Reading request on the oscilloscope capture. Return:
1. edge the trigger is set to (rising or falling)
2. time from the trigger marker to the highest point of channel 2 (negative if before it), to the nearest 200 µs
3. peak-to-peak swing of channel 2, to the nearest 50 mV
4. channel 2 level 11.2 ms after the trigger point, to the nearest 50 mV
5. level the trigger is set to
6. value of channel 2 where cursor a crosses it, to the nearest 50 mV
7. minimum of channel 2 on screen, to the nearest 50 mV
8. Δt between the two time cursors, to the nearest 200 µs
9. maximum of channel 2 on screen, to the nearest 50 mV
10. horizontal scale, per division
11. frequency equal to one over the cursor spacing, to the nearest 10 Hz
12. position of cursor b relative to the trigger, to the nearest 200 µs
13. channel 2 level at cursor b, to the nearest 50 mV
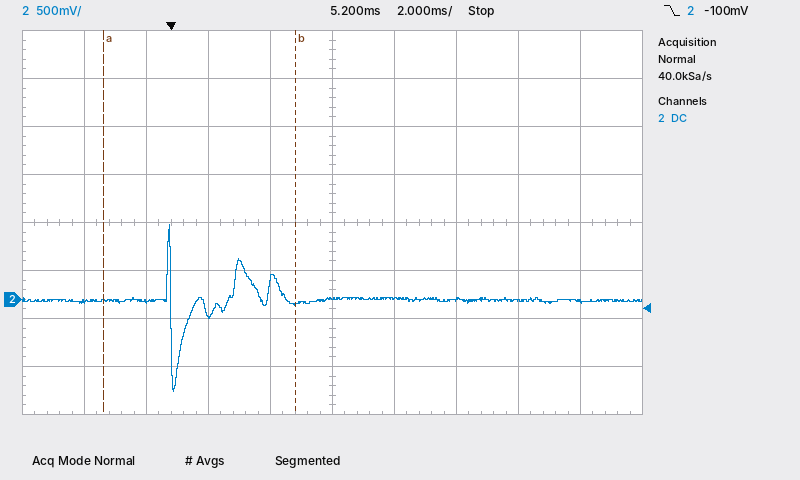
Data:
falling
0.0 ms
1.75 V
0 mV
-100 mV
0 mV
-950 mV
6.2 ms
800 mV
2 ms
160 Hz
+4.0 ms
-50 mV
